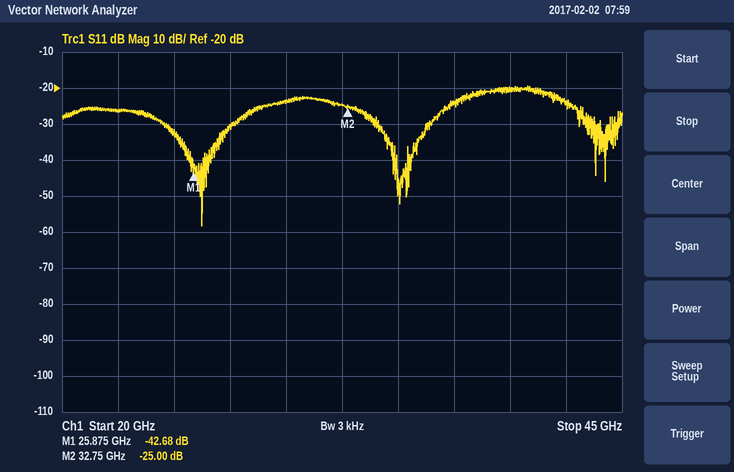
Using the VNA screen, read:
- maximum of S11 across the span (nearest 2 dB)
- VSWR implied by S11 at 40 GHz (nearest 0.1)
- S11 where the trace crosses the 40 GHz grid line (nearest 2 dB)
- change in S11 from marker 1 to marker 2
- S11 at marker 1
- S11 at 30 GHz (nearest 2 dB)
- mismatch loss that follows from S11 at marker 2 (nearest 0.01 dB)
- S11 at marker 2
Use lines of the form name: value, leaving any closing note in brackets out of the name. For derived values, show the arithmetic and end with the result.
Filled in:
maximum of S11 across the span: -20 dB
VSWR implied by S11 at 40 GHz: |Γ| = 10^(-20/20) = 0.1000; VSWR = (1 + 0.1000)/(1 − 0.1000) ≈ 1.2
S11 where the trace crosses the 40 GHz grid line: -20 dB
change in S11 from marker 1 to marker 2: -25 − (-42.68) = 17.68 dB
S11 at marker 1: -42.68 dB
S11 at 30 GHz: -24 dB
mismatch loss that follows from S11 at marker 2: −10 log10(1 − 10^(-25/10)) ≈ 0.01 dB
S11 at marker 2: -25.00 dB
